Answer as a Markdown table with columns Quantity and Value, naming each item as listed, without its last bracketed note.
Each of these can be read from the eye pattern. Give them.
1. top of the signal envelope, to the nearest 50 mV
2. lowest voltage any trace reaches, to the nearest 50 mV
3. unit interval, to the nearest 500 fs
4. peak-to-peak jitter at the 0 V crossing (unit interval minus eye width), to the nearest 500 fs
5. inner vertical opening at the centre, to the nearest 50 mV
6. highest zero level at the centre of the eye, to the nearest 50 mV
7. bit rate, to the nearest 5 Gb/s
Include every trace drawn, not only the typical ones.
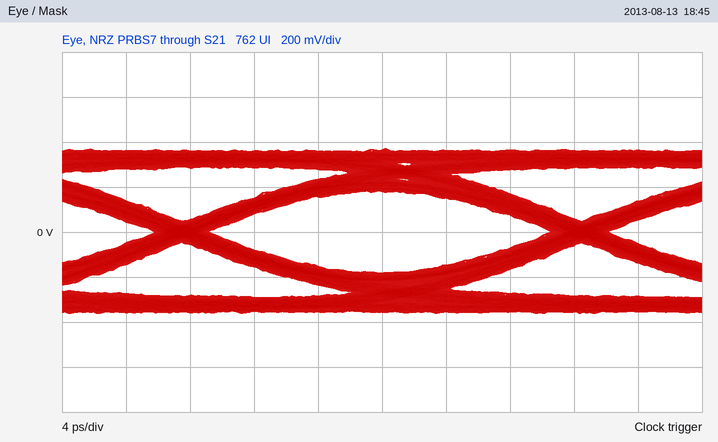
| Quantity | Value |
|---|---|
| top of the signal envelope, to the nearest 50 mV | 350 mV |
| lowest voltage any trace reaches, to the nearest 50 mV | -350 mV |
| unit interval, to the nearest 500 fs | 25.0 ps |
| peak-to-peak jitter at the 0 V crossing (unit interval minus eye width), to the nearest 500 fs | 3.5 ps |
| inner vertical opening at the centre, to the nearest 50 mV | 350 mV |
| highest zero level at the centre of the eye, to the nearest 50 mV | -200 mV |
| bit rate, to the nearest 5 Gb/s | 40 Gb/s |
